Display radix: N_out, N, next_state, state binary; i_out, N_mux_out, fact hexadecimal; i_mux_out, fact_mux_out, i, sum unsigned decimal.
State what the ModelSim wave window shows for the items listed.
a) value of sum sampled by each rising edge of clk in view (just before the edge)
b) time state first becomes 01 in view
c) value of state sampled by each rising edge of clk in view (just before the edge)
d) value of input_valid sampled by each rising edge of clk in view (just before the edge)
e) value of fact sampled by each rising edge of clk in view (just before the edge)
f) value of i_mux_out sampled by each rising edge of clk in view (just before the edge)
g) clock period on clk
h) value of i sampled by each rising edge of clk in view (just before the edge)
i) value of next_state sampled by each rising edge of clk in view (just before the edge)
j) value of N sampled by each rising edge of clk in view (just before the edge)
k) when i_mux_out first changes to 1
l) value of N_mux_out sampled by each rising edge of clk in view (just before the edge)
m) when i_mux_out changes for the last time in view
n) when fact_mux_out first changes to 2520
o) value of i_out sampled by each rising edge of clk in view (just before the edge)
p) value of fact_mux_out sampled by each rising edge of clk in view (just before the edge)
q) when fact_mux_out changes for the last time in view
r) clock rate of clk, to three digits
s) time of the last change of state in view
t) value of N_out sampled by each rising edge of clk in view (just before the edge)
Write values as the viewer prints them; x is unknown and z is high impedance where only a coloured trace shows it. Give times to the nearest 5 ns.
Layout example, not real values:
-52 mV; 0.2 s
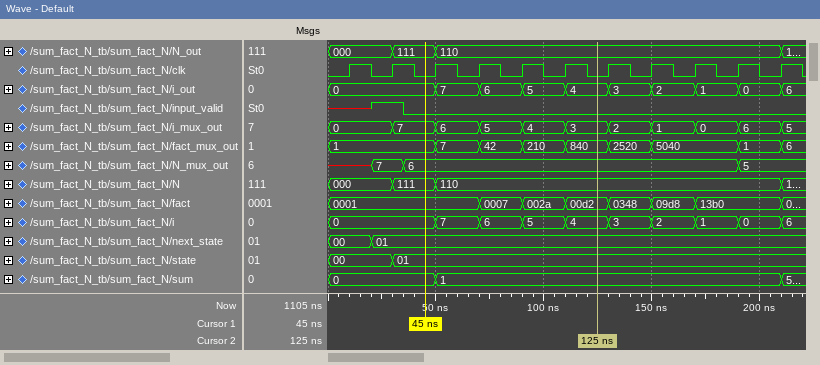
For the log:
0, 0, 0, 1, 1, 1, 1, 1, 1, 1, 1; 30 ns; 00, 00, 01, 01, 01, 01, 01, 01, 01, 01, 01; x 1 0 0 0 0 0 0 0 0 0; 0001, 0001, 0001, 0001, 0007, 002a, 00d2, 0348, 09d8, 13b0, 13b0; 0, 0, 7, 6, 5, 4, 3, 2, 1, 0, 6; 20 ns; 0, 0, 0, 7, 6, 5, 4, 3, 2, 1, 0; 00, 01, 01, 01, 01, 01, 01, 01, 01, 01, 01; 000, 000, 111, 110, 110, 110, 110, 110, 110, 110, 110; 150 ns; x, 7, 6, 6, 6, 6, 6, 6, 6, 6, 5; 210 ns; 130 ns; 0, 0, 0, 7, 6, 5, 4, 3, 2, 1, 0; 1, 1, 1, 7, 42, 210, 840, 2520, 5040, 5040, 1; 210 ns; 50.0 MHz; 30 ns; 000, 000, 111, 110, 110, 110, 110, 110, 110, 110, 110
